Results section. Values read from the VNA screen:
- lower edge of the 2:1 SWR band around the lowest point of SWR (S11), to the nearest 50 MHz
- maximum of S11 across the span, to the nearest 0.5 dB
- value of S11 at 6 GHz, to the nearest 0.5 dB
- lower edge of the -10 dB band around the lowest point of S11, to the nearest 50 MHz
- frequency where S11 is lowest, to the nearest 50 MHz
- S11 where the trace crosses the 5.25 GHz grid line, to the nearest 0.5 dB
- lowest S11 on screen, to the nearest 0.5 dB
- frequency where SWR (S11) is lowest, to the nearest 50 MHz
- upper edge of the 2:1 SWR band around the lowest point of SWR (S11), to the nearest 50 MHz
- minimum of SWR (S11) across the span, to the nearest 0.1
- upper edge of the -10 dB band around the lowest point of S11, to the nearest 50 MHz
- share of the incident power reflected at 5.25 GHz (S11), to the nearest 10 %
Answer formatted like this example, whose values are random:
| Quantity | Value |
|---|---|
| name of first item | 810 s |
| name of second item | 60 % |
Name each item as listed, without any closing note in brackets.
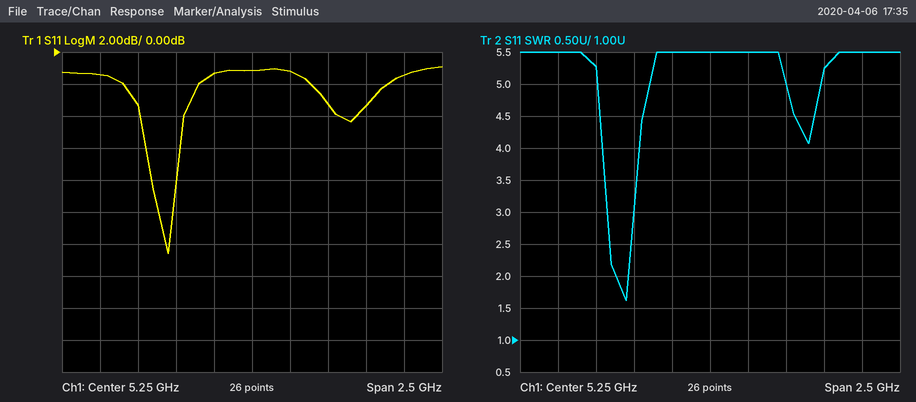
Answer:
| Quantity | Value |
|---|---|
| lower edge of the 2:1 SWR band around the lowest point of SWR (S11), to the nearest 50 MHz | 4.65 GHz |
| maximum of S11 across the span, to the nearest 0.5 dB | -1.0 dB |
| value of S11 at 6 GHz, to the nearest 0.5 dB | -3.5 dB |
| lower edge of the -10 dB band around the lowest point of S11, to the nearest 50 MHz | 4.65 GHz |
| frequency where S11 is lowest, to the nearest 50 MHz | 4.70 GHz |
| S11 where the trace crosses the 5.25 GHz grid line, to the nearest 0.5 dB | -1.0 dB |
| lowest S11 on screen, to the nearest 0.5 dB | -12.5 dB |
| frequency where SWR (S11) is lowest, to the nearest 50 MHz | 4.70 GHz |
| upper edge of the 2:1 SWR band around the lowest point of SWR (S11), to the nearest 50 MHz | 4.70 GHz |
| minimum of SWR (S11) across the span, to the nearest 0.1 | 1.6 |
| upper edge of the -10 dB band around the lowest point of S11, to the nearest 50 MHz | 4.75 GHz |
| share of the incident power reflected at 5.25 GHz (S11), to the nearest 10 % | 80 % |
